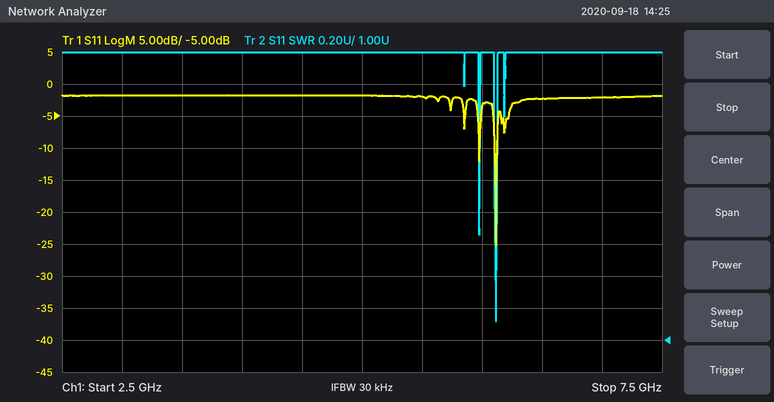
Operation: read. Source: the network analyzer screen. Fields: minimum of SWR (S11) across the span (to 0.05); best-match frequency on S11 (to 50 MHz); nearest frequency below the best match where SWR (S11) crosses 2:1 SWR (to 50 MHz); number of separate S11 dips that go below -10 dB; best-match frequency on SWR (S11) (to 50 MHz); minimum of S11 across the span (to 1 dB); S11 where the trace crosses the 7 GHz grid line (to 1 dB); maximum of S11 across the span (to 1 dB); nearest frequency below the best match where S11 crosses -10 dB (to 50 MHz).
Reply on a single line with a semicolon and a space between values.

1.10; 6.10 GHz; 6.10 GHz; 2; 6.10 GHz; -25 dB; -2 dB; -2 dB; 6.10 GHz
